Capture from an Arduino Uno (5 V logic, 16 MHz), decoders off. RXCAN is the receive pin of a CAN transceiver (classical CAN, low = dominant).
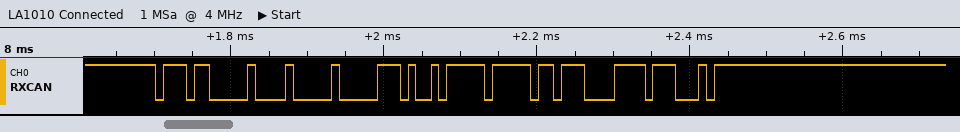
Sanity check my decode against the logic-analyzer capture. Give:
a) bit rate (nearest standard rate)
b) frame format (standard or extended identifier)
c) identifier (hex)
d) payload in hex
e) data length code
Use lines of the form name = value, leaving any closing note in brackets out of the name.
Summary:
bit rate = 100 kbit/s
frame format = standard
identifier = 0x760
payload in hex = 00 D2 FF F7
data length code = 4
